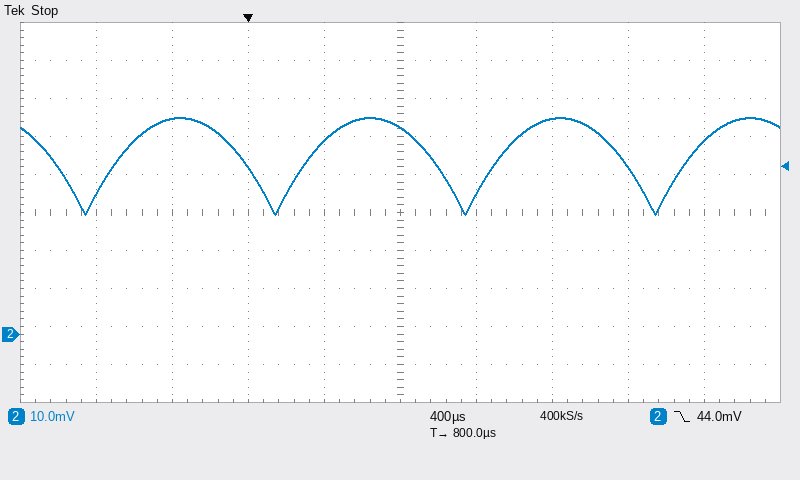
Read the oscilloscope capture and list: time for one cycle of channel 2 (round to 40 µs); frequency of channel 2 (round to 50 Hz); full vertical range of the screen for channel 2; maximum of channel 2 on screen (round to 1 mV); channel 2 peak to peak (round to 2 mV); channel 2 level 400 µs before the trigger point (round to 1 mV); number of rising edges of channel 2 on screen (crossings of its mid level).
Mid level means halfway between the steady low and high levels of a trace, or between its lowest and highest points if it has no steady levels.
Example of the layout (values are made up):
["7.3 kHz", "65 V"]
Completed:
["1.00 ms", "1.00 kHz", "100 mV", "57 mV", "26 mV", "57 mV", "4"]
